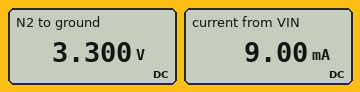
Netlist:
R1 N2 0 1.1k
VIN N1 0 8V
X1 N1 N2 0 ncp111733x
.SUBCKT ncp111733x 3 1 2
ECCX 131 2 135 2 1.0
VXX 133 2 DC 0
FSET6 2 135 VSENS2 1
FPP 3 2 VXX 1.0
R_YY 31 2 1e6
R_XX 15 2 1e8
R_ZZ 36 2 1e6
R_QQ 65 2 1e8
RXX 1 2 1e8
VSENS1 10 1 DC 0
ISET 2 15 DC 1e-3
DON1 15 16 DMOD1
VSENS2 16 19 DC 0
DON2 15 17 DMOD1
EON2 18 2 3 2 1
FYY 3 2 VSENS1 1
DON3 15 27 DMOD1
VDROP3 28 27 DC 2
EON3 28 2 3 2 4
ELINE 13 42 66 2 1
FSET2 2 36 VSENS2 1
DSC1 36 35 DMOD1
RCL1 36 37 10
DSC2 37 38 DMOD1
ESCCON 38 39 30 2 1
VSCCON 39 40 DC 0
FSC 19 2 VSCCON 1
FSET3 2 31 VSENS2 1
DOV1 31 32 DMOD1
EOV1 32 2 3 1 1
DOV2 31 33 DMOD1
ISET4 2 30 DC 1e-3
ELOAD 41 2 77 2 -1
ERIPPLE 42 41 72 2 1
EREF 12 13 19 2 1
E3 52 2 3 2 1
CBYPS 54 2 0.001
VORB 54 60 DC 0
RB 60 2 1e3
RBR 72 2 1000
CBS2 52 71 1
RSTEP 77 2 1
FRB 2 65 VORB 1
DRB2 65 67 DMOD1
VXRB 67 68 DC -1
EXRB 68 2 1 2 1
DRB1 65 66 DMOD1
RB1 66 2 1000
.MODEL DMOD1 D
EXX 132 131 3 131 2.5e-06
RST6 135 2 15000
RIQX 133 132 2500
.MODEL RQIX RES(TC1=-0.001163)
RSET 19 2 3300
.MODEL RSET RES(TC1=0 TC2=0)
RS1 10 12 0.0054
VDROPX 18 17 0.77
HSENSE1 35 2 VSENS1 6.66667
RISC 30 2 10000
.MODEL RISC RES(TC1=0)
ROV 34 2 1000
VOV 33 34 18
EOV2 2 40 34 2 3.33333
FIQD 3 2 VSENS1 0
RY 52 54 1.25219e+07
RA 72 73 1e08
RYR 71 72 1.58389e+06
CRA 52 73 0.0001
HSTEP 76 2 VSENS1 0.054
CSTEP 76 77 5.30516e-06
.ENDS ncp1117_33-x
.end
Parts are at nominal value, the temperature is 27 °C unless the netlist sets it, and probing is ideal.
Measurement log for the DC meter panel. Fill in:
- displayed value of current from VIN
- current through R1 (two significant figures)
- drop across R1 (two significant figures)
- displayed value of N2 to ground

9.00 mA
3.0 mA
3.3 V
3.300 V
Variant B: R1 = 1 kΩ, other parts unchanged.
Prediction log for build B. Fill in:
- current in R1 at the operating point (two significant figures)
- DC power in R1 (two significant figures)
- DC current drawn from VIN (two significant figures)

3.3 mA
11 mW
9.3 mA
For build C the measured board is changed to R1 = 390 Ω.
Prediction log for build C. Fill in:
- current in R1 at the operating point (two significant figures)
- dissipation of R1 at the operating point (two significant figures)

8.5 mA
28 mW
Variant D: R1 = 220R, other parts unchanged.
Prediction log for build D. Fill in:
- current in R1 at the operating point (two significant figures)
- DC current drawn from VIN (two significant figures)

15 mA
21 mA
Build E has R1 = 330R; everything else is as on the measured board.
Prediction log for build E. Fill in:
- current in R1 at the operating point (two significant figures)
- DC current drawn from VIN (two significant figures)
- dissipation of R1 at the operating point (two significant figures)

10 mA
16 mA
33 mW
